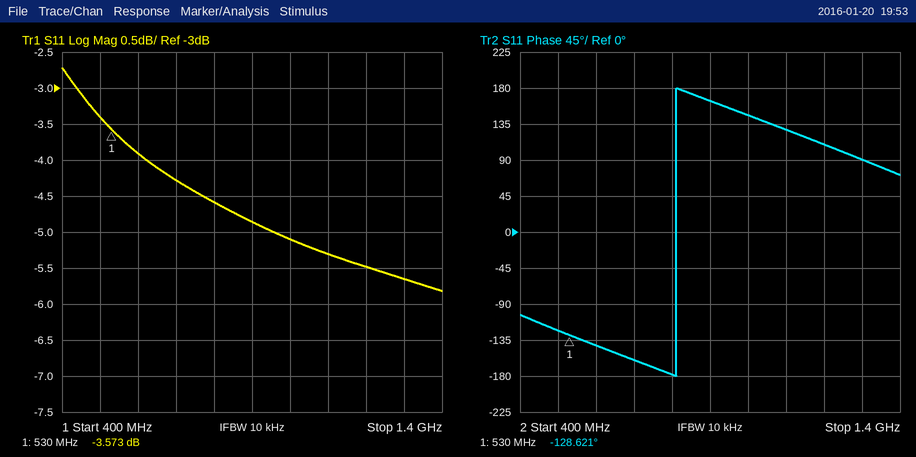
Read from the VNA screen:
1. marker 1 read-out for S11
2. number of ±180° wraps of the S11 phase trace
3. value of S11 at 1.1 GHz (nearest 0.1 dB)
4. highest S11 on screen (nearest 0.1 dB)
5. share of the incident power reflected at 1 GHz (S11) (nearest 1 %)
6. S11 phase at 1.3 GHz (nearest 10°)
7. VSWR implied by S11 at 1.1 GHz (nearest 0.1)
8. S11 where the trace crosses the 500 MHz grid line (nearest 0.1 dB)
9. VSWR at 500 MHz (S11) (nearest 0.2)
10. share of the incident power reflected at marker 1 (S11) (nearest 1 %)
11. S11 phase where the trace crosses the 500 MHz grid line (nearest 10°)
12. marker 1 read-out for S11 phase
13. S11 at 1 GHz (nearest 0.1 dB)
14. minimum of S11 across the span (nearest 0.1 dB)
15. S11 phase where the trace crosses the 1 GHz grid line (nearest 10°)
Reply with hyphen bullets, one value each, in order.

- -3.573 dB
- 1
- -5.3 dB
- -2.7 dB
- 31 %
- 90°
- 3.4
- -3.4 dB
- 5.2
- 44 %
- -120°
- -128.621°
- -5.1 dB
- -5.8 dB
- 150°
